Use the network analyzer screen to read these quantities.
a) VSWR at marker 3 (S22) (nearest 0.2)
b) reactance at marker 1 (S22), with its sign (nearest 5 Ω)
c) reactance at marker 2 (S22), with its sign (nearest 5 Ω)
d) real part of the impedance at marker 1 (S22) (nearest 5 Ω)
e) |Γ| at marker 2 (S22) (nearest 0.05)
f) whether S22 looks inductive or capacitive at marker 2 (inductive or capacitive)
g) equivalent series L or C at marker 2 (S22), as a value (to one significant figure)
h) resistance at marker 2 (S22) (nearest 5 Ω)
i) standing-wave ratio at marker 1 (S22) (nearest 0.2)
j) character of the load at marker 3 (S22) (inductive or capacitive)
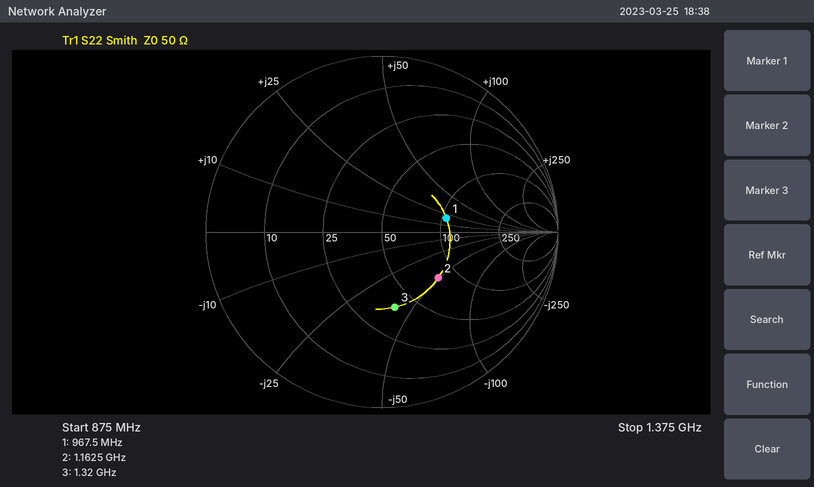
2.6
+20 Ω
-50 Ω
105 Ω
0.40
capacitive
3 pF
80 Ω
2.2
capacitive
